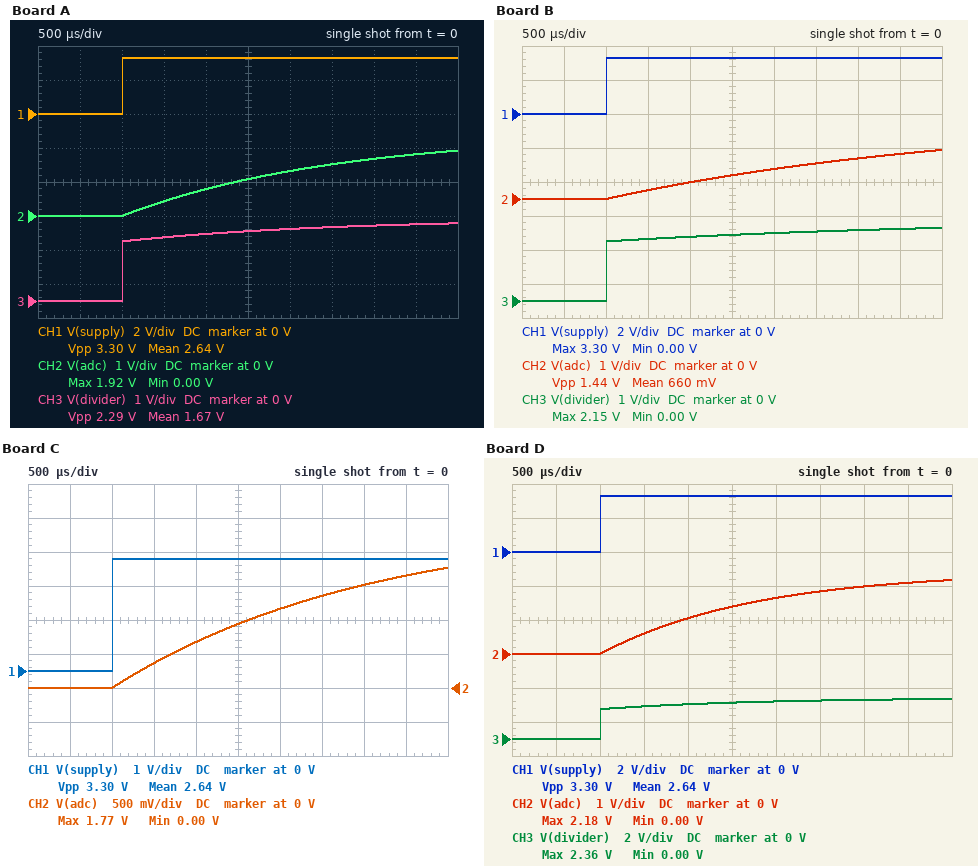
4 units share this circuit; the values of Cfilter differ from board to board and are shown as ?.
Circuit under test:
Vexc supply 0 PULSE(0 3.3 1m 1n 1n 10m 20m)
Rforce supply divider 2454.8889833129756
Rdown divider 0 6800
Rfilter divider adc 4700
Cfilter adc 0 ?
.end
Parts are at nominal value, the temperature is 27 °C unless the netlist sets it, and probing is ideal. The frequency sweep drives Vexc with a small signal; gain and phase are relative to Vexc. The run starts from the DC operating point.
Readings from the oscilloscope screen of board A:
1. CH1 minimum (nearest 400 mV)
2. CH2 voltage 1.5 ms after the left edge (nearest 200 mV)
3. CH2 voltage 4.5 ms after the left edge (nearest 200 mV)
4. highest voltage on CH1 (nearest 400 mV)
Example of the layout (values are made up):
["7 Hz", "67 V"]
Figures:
["0 V", "400 mV", "1.8 V", "3.2 V"]
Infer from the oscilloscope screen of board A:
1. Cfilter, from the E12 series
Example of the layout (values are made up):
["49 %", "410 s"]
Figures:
["390 nF"]
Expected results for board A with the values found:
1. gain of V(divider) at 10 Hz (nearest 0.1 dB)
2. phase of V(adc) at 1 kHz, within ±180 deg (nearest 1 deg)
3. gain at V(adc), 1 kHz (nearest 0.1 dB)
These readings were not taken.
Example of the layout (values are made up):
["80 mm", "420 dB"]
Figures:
["-2.7 dB", "-86 deg", "-26.7 dB"]
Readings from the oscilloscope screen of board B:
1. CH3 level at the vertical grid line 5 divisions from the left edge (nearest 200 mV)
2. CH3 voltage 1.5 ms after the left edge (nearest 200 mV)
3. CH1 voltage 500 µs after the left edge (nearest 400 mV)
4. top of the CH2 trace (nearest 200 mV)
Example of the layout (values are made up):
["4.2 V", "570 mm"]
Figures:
["2.0 V", "1.8 V", "0 V", "1.4 V"]
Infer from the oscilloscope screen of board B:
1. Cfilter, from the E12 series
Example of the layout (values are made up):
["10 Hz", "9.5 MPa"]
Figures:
["680 nF"]
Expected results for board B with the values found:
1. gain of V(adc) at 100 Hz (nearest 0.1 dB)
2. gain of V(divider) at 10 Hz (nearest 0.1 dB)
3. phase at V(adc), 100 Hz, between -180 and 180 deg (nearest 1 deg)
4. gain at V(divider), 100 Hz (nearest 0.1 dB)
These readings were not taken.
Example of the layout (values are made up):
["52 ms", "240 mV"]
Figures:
["-12.1 dB", "-2.8 dB", "-70 deg", "-5.1 dB"]
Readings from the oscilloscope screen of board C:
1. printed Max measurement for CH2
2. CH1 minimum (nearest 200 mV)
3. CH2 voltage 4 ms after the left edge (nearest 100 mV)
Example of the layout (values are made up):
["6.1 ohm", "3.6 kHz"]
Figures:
["1.77 V", "0 V", "1.5 V"]
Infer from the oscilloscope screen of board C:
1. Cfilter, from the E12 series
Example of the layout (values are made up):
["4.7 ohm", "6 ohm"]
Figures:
["470 nF"]
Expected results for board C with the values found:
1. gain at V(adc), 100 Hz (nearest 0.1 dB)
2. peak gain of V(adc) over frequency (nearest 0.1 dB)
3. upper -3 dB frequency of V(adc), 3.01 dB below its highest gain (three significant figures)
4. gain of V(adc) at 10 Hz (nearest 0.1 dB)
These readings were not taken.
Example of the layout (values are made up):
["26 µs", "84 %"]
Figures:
["-9.4 dB", "-2.7 dB", "52.1 Hz", "-2.8 dB"]
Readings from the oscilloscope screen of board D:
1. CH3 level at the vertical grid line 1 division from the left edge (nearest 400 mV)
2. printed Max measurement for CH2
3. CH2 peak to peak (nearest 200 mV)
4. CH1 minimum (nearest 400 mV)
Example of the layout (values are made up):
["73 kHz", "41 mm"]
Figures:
["0 V", "2.18 V", "2.2 V", "0 V"]
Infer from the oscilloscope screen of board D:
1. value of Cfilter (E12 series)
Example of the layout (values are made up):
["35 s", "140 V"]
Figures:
["270 nF"]
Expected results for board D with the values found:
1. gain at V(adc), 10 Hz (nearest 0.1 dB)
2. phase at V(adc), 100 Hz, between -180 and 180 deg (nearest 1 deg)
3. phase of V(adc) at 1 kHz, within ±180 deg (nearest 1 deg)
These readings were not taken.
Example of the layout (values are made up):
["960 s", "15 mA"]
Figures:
["-2.7 dB", "-48 deg", "-85 deg"]
